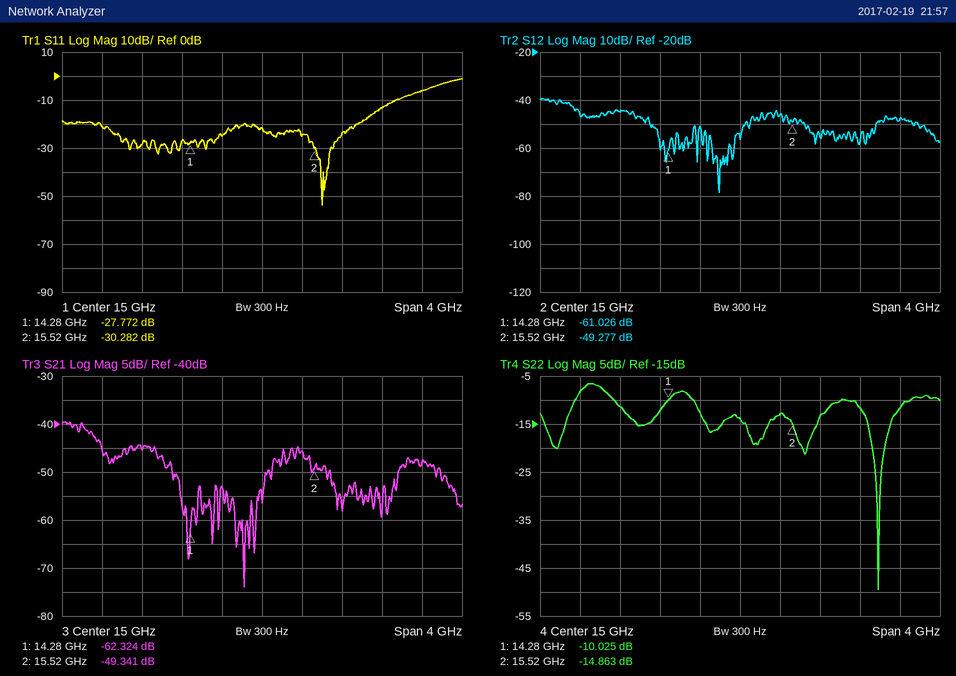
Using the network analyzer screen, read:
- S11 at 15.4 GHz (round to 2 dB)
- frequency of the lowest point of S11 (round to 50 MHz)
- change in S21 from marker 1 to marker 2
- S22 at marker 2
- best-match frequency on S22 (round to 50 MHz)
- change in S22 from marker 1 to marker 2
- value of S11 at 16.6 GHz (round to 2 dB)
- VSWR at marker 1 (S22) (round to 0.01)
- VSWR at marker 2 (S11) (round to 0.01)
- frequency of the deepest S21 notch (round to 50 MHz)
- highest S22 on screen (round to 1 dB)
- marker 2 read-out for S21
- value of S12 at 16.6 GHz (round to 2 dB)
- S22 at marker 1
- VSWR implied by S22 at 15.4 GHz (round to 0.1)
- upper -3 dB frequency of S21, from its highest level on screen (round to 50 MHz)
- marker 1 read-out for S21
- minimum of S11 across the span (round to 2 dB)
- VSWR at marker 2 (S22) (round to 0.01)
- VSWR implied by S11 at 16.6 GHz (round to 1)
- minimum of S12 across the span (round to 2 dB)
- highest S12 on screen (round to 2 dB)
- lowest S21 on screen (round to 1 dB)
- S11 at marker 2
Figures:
-24 dB
15.60 GHz
12.983 dB
-14.863 dB
16.40 GHz
-4.838 dB
-6 dB
1.92
1.06
14.80 GHz
-7 dB
-49.341 dB
-48 dB
-10.025 dB
1.6
13.30 GHz
-62.324 dB
-54 dB
1.44
3
-78 dB
-40 dB
-74 dB
-30.282 dB
